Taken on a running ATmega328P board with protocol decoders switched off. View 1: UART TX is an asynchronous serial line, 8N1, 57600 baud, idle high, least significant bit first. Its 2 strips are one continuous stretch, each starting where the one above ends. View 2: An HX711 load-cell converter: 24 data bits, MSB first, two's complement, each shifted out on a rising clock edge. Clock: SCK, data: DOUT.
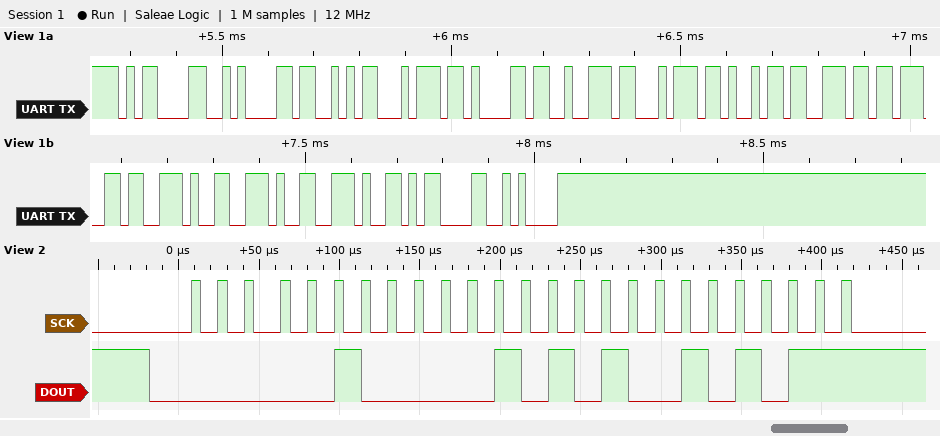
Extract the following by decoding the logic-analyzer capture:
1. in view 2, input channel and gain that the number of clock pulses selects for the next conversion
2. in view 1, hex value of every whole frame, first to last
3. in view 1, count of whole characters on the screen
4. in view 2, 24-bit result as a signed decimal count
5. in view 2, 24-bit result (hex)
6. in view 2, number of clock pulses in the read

channel A, gain 128
0x0D 0x0A 0x53 0x74 0x61 0x72 0x74 0x69 0x6E 0x67 0x2E 0x2E 0x2E 0x0D 0x0A
15
267563
0x04152B
25
